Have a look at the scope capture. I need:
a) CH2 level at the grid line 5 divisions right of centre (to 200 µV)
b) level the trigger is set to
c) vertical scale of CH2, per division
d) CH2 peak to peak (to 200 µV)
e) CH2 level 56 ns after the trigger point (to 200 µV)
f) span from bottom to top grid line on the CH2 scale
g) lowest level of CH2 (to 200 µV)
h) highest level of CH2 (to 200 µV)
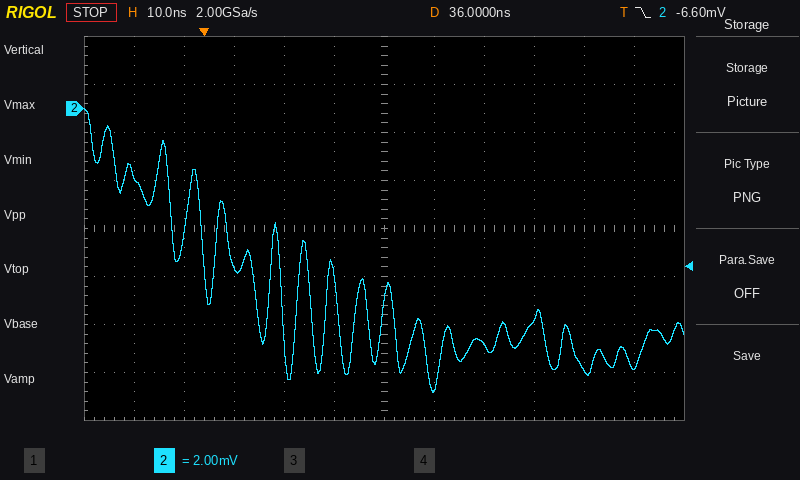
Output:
-10.8 mV
-6.60 mV
2 mV
11.8 mV
-9.8 mV
16 mV
-11.8 mV
0.0 mV
